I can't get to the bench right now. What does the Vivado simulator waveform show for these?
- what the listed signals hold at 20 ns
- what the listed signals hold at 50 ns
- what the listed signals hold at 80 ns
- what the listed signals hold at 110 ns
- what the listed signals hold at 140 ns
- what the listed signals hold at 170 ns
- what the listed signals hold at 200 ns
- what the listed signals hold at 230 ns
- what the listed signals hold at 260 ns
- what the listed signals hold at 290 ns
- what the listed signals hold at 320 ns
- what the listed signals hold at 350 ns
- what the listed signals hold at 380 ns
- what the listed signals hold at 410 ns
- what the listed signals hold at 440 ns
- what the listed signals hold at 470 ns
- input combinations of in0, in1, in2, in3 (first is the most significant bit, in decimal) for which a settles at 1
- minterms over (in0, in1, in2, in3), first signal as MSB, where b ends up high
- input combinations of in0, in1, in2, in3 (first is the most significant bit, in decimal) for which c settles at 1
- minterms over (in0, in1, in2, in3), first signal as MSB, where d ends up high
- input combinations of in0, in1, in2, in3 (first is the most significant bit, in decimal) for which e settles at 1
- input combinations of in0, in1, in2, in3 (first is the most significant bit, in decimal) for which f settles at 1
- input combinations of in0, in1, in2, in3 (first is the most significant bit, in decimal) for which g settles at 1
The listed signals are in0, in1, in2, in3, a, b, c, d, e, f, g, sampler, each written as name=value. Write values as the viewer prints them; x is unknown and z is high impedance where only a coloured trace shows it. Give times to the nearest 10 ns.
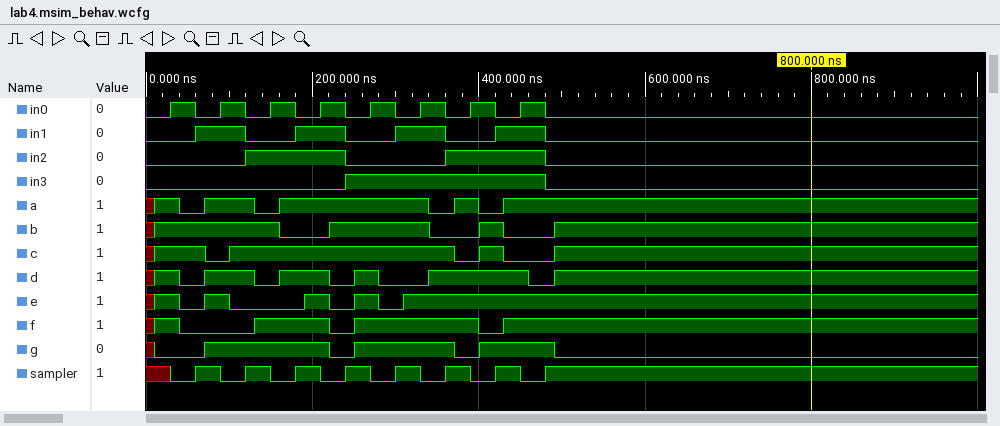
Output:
in0=0, in1=0, in2=0, in3=0, a=1, b=1, c=1, d=1, e=1, f=1, g=0, sampler=x
in0=1, in1=0, in2=0, in3=0, a=0, b=1, c=1, d=0, e=0, f=0, g=0, sampler=0
in0=0, in1=1, in2=0, in3=0, a=1, b=1, c=0, d=1, e=1, f=0, g=1, sampler=1
in0=1, in1=1, in2=0, in3=0, a=1, b=1, c=1, d=1, e=0, f=0, g=1, sampler=0
in0=0, in1=0, in2=1, in3=0, a=0, b=1, c=1, d=0, e=0, f=1, g=1, sampler=1
in0=1, in1=0, in2=1, in3=0, a=1, b=0, c=1, d=1, e=0, f=1, g=1, sampler=0
in0=0, in1=1, in2=1, in3=0, a=1, b=0, c=1, d=1, e=1, f=1, g=1, sampler=1
in0=1, in1=1, in2=1, in3=0, a=1, b=1, c=1, d=0, e=0, f=0, g=0, sampler=0
in0=0, in1=0, in2=0, in3=1, a=1, b=1, c=1, d=1, e=1, f=1, g=1, sampler=1
in0=1, in1=0, in2=0, in3=1, a=1, b=1, c=1, d=0, e=0, f=1, g=1, sampler=0
in0=0, in1=1, in2=0, in3=1, a=1, b=1, c=1, d=0, e=1, f=1, g=1, sampler=1
in0=1, in1=1, in2=0, in3=1, a=0, b=0, c=1, d=1, e=1, f=1, g=1, sampler=0
in0=0, in1=0, in2=1, in3=1, a=1, b=0, c=0, d=1, e=1, f=1, g=0, sampler=1
in0=1, in1=0, in2=1, in3=1, a=0, b=1, c=1, d=1, e=1, f=0, g=1, sampler=0
in0=0, in1=1, in2=1, in3=1, a=1, b=0, c=0, d=1, e=1, f=1, g=1, sampler=1
in0=1, in1=1, in2=1, in3=1, a=1, b=0, c=0, d=0, e=1, f=1, g=1, sampler=0
0, 1, 3, 4, 5, 6, 7, 9, 10, 12, 14, 15
0, 1, 2, 4, 5, 8, 9, 11, 12, 14
0, 1, 2, 5, 6, 8, 9, 10, 11, 12, 13, 14
0, 1, 3, 4, 6, 7, 10, 11, 12, 13
0, 1, 3, 4, 5, 6, 7, 11, 13, 15
0, 1, 2, 3, 5, 6, 7, 9, 10, 13, 15
1, 2, 4, 5, 6, 7, 9, 10, 11, 12, 13, 15
